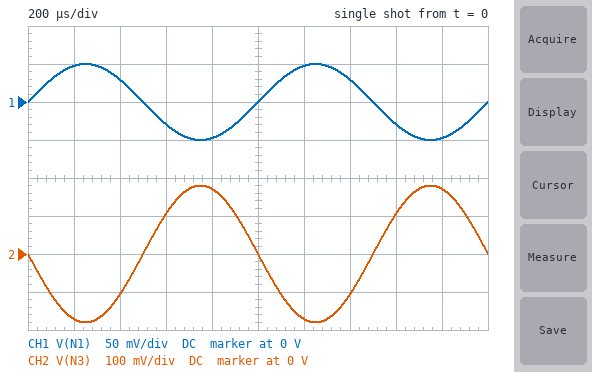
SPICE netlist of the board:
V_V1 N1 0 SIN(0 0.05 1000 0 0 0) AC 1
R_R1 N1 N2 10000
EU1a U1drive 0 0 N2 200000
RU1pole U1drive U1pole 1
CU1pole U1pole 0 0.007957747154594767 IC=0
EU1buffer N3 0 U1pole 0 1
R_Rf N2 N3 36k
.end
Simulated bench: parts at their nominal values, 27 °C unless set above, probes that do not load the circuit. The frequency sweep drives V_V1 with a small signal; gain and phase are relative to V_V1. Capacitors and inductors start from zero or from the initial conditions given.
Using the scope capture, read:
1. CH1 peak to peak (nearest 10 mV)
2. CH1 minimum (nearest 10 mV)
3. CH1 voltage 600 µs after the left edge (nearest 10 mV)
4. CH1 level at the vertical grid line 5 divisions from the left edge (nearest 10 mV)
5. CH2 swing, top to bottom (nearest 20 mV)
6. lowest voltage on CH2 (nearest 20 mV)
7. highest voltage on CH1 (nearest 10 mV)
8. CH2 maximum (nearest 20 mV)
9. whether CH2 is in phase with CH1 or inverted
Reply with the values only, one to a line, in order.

100 mV
-50 mV
-30 mV
0 V
360 mV
-180 mV
50 mV
180 mV
inverted
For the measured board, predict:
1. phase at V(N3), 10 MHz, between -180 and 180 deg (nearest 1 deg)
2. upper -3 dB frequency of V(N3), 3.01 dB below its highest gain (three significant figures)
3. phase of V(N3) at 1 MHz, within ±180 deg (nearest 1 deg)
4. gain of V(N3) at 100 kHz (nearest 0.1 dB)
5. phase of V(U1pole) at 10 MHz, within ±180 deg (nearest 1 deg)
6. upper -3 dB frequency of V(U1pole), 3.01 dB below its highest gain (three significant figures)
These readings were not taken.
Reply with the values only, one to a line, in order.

95 deg
870 kHz
131 deg
11.1 dB
95 deg
870 kHz
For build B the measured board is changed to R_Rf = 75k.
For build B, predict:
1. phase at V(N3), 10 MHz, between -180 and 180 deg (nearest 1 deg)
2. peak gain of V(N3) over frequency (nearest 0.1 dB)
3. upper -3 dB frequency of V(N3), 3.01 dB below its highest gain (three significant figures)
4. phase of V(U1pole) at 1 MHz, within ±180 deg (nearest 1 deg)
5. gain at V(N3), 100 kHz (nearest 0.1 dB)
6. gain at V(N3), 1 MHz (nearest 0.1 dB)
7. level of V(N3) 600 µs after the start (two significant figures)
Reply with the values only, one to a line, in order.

93 deg
17.5 dB
471 kHz
115 deg
17.3 dB
10.1 dB
220 mV
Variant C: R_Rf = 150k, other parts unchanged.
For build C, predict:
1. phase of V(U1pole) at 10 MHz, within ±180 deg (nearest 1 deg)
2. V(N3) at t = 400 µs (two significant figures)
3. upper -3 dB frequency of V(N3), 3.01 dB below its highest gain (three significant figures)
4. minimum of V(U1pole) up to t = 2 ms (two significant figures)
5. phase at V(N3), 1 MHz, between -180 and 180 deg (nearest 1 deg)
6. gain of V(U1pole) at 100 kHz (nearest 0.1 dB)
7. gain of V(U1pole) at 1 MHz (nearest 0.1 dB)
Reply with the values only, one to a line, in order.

91 deg
-440 mV
250 kHz
-750 mV
104 deg
22.9 dB
11.2 dB
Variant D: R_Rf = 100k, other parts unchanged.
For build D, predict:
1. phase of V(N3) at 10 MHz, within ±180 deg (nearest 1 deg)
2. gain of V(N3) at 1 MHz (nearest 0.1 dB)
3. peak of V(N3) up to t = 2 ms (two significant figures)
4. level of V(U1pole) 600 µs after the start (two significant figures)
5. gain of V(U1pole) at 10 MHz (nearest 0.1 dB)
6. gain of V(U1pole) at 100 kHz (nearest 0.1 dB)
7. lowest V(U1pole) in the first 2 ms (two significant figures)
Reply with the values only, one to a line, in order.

92 deg
10.7 dB
500 mV
290 mV
-8.8 dB
19.7 dB
-500 mV
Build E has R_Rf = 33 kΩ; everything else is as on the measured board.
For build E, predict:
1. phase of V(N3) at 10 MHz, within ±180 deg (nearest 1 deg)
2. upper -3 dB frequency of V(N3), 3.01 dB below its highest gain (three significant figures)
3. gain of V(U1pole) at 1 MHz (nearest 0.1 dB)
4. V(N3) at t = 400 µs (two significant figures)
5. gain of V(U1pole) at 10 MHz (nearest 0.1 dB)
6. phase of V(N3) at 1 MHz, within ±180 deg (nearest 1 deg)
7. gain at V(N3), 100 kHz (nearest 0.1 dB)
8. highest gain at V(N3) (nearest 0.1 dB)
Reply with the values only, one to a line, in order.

95 deg
930 kHz
7.0 dB
-97 mV
-10.3 dB
133 deg
10.3 dB
10.4 dB
